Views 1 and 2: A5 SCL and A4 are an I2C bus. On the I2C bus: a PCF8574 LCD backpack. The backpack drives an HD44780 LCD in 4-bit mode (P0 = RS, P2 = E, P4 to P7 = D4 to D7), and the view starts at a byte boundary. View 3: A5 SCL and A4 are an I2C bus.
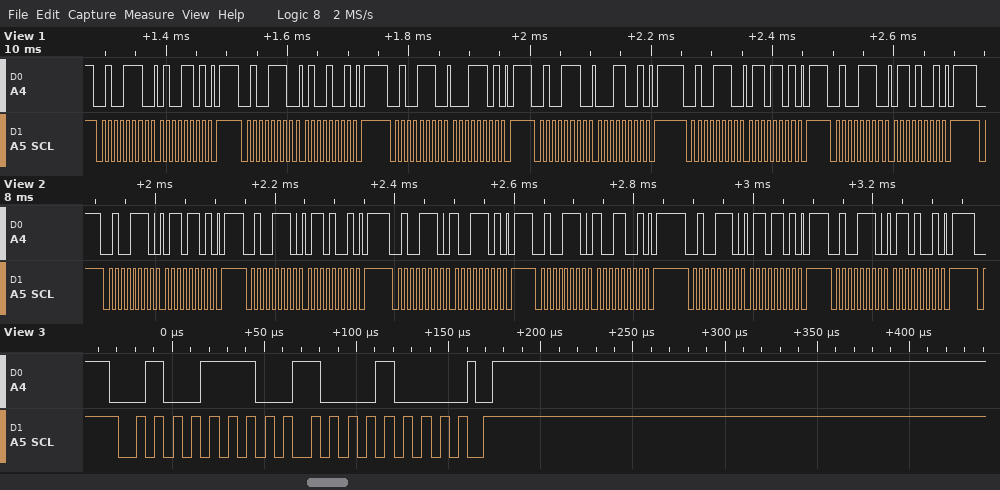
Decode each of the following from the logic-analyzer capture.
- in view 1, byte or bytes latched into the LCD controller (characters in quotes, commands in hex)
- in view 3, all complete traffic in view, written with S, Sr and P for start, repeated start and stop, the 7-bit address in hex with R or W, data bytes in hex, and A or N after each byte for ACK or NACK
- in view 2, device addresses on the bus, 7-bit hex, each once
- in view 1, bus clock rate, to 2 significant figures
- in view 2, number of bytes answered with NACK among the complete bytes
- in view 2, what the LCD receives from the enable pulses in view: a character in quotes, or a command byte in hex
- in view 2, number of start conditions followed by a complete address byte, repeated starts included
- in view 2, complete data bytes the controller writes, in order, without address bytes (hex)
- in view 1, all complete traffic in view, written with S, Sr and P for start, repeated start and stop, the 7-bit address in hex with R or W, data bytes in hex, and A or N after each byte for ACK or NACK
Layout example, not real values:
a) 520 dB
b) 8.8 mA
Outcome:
a) 'A'
b) S 27W A 88 A P
c) 0x27
d) 100 kHz
e) 0
f) 'i'
g) 6
h) 6D 69 9D 99 6D 69
i) S 27W A 4D A P S 27W A 49 A P S 27W A 1D A P S 27W A 19 A P S 27W A 6D A P S 27W A 69 A P
